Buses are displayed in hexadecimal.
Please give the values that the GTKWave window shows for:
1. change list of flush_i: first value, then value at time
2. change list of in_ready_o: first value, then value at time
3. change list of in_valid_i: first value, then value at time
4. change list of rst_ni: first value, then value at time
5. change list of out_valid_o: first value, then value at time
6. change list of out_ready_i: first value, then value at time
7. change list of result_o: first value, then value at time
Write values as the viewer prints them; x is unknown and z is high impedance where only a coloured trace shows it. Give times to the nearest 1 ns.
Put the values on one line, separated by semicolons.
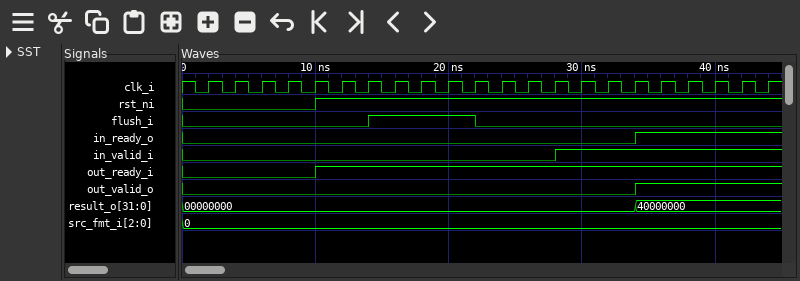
0, 1 at 14 ns, 0 at 22 ns; 0, 1 at 34 ns; 0, 1 at 28 ns; 0, 1 at 10 ns; 0, 1 at 34 ns; 0, 1 at 10 ns; 00000000, 40000000 at 34 ns
